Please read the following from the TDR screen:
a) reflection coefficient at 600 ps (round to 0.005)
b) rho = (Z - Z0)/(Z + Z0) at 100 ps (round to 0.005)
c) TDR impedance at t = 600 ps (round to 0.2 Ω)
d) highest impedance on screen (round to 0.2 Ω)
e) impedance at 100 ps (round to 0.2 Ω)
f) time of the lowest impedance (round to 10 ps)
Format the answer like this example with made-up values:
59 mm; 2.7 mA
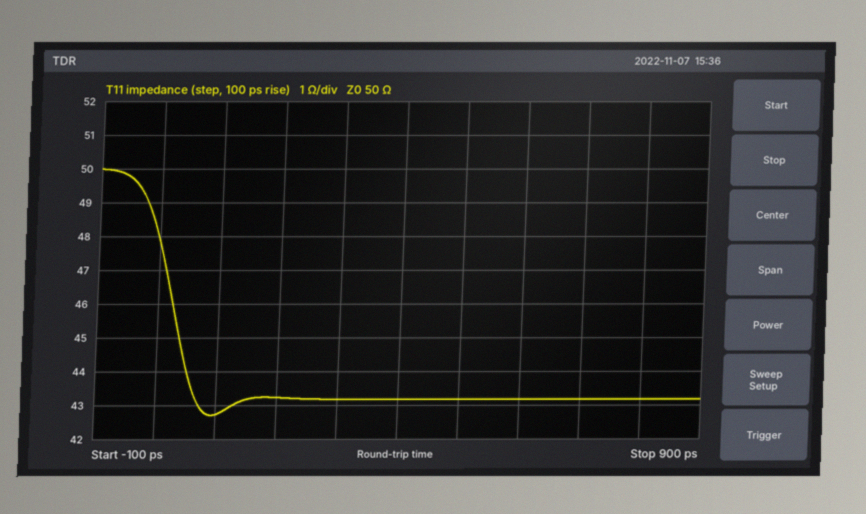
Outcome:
-0.075; -0.080; 43.2 Ω; 50.0 Ω; 42.8 Ω; 90 ps
